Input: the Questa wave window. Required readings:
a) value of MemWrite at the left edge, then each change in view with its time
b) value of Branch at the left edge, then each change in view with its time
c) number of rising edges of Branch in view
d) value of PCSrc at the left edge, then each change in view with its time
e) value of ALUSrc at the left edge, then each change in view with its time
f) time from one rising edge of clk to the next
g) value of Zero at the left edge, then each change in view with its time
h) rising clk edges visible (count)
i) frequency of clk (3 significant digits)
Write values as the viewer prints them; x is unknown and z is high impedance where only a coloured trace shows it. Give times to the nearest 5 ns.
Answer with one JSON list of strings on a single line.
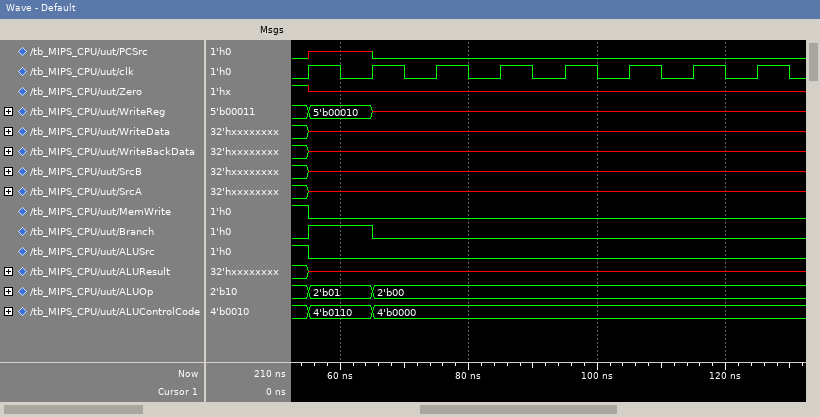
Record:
["1, 0 at 55 ns", "0, 1 at 55 ns, 0 at 65 ns", "1", "0, x at 55 ns, 0 at 65 ns", "1, 0 at 55 ns", "10 ns", "1, x at 55 ns", "8", "100 MHz"]
